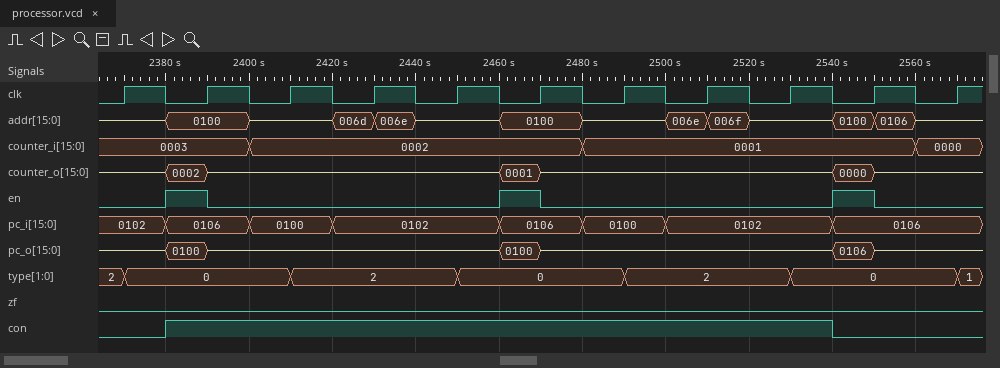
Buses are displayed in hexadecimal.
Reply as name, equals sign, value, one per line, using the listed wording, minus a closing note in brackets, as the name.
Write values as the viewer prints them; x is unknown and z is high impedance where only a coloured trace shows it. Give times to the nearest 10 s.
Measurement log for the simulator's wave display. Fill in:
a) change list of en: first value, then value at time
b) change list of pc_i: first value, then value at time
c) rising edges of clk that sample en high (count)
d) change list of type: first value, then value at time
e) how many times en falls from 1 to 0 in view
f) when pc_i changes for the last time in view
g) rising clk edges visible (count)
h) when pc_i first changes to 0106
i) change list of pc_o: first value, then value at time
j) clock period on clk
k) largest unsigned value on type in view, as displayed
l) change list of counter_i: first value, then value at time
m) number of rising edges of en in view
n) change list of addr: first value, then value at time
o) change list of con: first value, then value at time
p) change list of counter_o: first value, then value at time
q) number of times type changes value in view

change list of en: first value, then value at time = 0, 1 at 2380 s, 0 at 2390 s, 1 at 2460 s, 0 at 2470 s, 1 at 2540 s, 0 at 2550 s
change list of pc_i: first value, then value at time = 0102, 0106 at 2380 s, 0100 at 2400 s, 0102 at 2420 s, 0106 at 2460 s, 0100 at 2480 s, 0102 at 2500 s, 0106 at 2540 s
rising edges of clk that sample en high = 3
change list of type: first value, then value at time = 2, 0 at 2370 s, 2 at 2410 s, 0 at 2450 s, 2 at 2490 s, 0 at 2530 s, 1 at 2570 s
how many times en falls from 1 to 0 in view = 3
when pc_i changes for the last time in view = 2540 s
rising clk edges visible = 11
when pc_i first changes to 0106 = 2380 s
change list of pc_o: first value, then value at time = z, 0100 at 2380 s, z at 2390 s, 0100 at 2460 s, z at 2470 s, 0106 at 2540 s, z at 2550 s
clock period on clk = 20 s
largest unsigned value on type in view, as displayed = 2
change list of counter_i: first value, then value at time = 0003, 0002 at 2400 s, 0001 at 2480 s, 0000 at 2560 s
number of rising edges of en in view = 3
change list of addr: first value, then value at time = z, 0100 at 2380 s, z at 2400 s, 006d at 2420 s, 006e at 2430 s, z at 2440 s, 0100 at 2460 s, z at 2480 s, 006e at 2500 s, 006f at 2510 s, z at 2520 s, 0100 at 2540 s, 0106 at 2550 s, z at 2560 s
change list of con: first value, then value at time = 0, 1 at 2380 s, 0 at 2540 s
change list of counter_o: first value, then value at time = z, 0002 at 2380 s, z at 2390 s, 0001 at 2460 s, z at 2470 s, 0000 at 2540 s, z at 2550 s
number of times type changes value in view = 6
